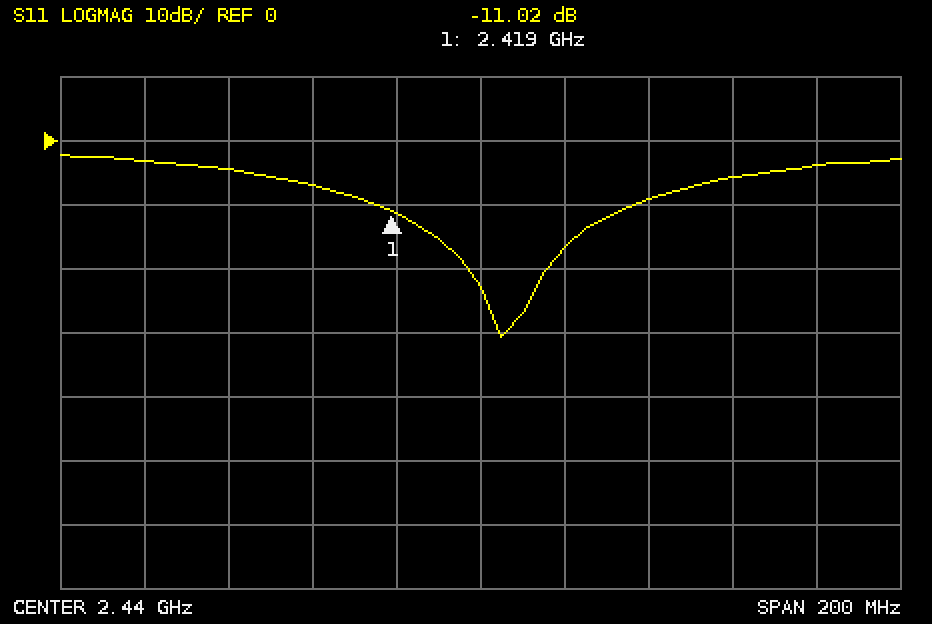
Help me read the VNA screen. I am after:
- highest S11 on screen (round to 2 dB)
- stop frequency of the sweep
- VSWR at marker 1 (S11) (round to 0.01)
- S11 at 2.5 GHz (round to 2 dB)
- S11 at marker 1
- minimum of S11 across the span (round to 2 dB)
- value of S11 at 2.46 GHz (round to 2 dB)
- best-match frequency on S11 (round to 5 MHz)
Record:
-2 dB
2.54 GHz
1.78
-6 dB
-11.02 dB
-30 dB
-16 dB
2.445 GHz
